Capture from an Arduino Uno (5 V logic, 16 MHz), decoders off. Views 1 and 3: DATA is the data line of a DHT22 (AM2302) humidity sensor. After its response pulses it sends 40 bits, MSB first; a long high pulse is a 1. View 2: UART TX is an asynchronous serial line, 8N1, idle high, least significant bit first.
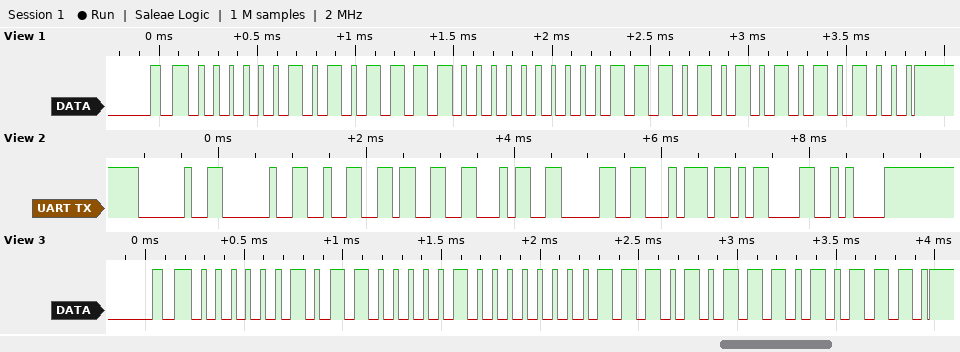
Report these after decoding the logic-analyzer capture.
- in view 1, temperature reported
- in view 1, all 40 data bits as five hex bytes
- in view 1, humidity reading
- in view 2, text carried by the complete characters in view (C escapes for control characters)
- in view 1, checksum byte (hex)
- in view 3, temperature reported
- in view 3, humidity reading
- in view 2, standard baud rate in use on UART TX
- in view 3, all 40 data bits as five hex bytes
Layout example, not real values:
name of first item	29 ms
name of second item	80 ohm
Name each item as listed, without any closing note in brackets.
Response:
in view 1, temperature reported	23.4 °C
in view 1, all 40 data bits as five hex bytes	02 BC 00 EA A8
in view 1, humidity reading	70.0 %
in view 2, text carried by the complete characters in view	"  2340t\r\n"
in view 1, checksum byte	0xA8
in view 3, temperature reported	23.5 °C
in view 3, humidity reading	70.5 %
in view 2, standard baud rate in use on UART TX	9600 baud
in view 3, all 40 data bits as five hex bytes	02 C1 00 EB AE
